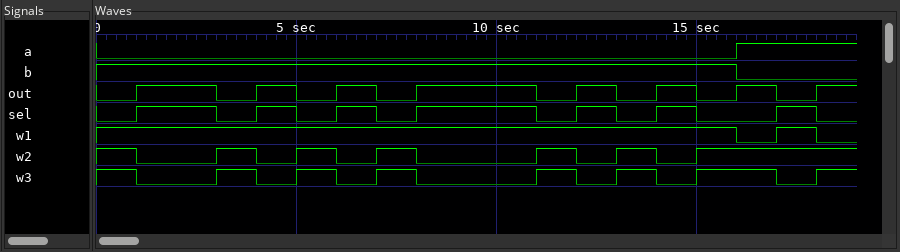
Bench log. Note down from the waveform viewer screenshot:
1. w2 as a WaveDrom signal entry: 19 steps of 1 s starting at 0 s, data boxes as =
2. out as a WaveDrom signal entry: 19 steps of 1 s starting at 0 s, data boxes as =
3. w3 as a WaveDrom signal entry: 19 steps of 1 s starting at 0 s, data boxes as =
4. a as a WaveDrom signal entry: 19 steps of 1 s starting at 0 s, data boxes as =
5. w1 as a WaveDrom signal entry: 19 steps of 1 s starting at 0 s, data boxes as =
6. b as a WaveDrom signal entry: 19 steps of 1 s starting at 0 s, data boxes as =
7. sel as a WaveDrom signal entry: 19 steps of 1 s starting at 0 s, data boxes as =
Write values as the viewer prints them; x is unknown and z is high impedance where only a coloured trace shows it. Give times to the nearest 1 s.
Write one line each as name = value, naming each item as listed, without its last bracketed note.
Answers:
w2 as a WaveDrom signal entry: 19 steps of 1 s starting at 0 s, data boxes as = = {name: 'w2', wave: '10.101010..10101...'}
out as a WaveDrom signal entry: 19 steps of 1 s starting at 0 s, data boxes as = = {name: 'out', wave: '01.010101..01010101'}
w3 as a WaveDrom signal entry: 19 steps of 1 s starting at 0 s, data boxes as = = {name: 'w3', wave: '10.101010..10101.01'}
a as a WaveDrom signal entry: 19 steps of 1 s starting at 0 s, data boxes as = = {name: 'a', wave: '0...............1..'}
w1 as a WaveDrom signal entry: 19 steps of 1 s starting at 0 s, data boxes as = = {name: 'w1', wave: '1...............010'}
b as a WaveDrom signal entry: 19 steps of 1 s starting at 0 s, data boxes as = = {name: 'b', wave: '1...............0..'}
sel as a WaveDrom signal entry: 19 steps of 1 s starting at 0 s, data boxes as = = {name: 'sel', wave: '01.010101..01010.10'}
